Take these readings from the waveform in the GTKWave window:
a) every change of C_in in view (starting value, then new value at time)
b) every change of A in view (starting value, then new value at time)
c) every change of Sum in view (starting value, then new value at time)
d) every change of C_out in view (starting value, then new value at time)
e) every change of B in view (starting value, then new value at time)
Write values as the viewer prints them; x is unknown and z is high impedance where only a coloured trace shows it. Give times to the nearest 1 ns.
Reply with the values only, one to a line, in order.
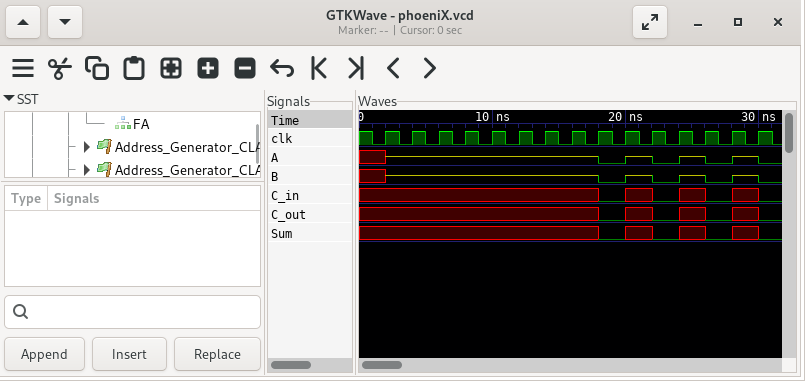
x, 0 at 18 ns, x at 20 ns, 0 at 22 ns, x at 24 ns, 0 at 26 ns, x at 28 ns, 0 at 30 ns
x, z at 2 ns, 0 at 18 ns, z at 20 ns, 0 at 22 ns, z at 24 ns, 0 at 26 ns, z at 28 ns, 0 at 30 ns
x, 0 at 18 ns, x at 20 ns, 0 at 22 ns, x at 24 ns, 0 at 26 ns, x at 28 ns, 0 at 30 ns
x, 0 at 18 ns, x at 20 ns, 0 at 22 ns, x at 24 ns, 0 at 26 ns, x at 28 ns, 0 at 30 ns
x, z at 2 ns, 0 at 18 ns, z at 20 ns, 0 at 22 ns, z at 24 ns, 0 at 26 ns, z at 28 ns, 0 at 30 ns
